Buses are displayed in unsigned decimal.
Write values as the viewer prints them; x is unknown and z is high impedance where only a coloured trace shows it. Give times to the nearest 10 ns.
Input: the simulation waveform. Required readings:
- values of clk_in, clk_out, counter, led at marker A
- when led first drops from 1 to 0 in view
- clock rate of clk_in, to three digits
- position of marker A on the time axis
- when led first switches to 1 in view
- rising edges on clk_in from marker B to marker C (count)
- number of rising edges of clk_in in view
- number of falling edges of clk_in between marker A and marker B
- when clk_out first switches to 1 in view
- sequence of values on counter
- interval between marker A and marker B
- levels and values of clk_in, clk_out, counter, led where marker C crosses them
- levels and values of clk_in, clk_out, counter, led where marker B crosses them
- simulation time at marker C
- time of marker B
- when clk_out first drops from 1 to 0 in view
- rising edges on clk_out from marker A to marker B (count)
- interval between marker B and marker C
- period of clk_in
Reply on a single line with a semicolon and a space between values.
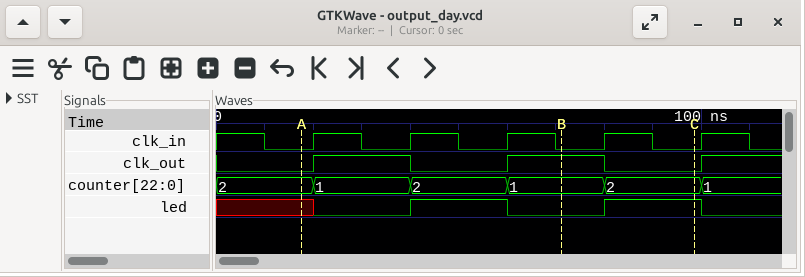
clk_in=0, clk_out=0, counter=2, led=x; 60 ns; 50.0 MHz; 20 ns; 40 ns; 1; 5; 3; 20 ns; 2, 1, 2, 1, 2, 1; 50 ns; clk_in=0, clk_out=0, counter=2, led=1; clk_in=0, clk_out=1, counter=1, led=0; 100 ns; 70 ns; 40 ns; 2; 30 ns; 20 ns
